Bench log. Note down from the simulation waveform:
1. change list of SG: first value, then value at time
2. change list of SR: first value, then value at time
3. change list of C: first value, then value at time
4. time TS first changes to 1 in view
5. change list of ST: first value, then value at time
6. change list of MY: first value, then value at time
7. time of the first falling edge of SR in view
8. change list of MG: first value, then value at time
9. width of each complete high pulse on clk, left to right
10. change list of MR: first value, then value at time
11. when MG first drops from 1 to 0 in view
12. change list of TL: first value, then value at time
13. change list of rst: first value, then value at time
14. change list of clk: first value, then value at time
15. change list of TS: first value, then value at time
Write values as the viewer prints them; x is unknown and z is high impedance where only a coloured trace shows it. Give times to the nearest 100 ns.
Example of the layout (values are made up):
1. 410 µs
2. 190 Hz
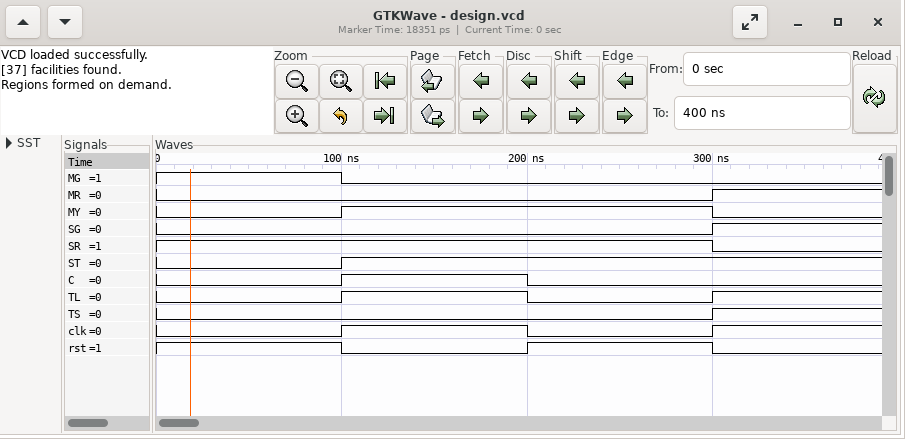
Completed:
1. 0, 1 at 300 ns
2. 1, 0 at 300 ns
3. 0, 1 at 100 ns, 0 at 200 ns
4. 300 ns
5. 0, 1 at 100 ns
6. 0, 1 at 100 ns, 0 at 300 ns
7. 300 ns
8. 1, 0 at 100 ns
9. 100 ns
10. 0, 1 at 300 ns
11. 100 ns
12. 0, 1 at 100 ns, 0 at 200 ns, 1 at 300 ns
13. 1, 0 at 100 ns, 1 at 200 ns, 0 at 300 ns
14. 0, 1 at 100 ns, 0 at 200 ns, 1 at 300 ns
15. 0, 1 at 300 ns
